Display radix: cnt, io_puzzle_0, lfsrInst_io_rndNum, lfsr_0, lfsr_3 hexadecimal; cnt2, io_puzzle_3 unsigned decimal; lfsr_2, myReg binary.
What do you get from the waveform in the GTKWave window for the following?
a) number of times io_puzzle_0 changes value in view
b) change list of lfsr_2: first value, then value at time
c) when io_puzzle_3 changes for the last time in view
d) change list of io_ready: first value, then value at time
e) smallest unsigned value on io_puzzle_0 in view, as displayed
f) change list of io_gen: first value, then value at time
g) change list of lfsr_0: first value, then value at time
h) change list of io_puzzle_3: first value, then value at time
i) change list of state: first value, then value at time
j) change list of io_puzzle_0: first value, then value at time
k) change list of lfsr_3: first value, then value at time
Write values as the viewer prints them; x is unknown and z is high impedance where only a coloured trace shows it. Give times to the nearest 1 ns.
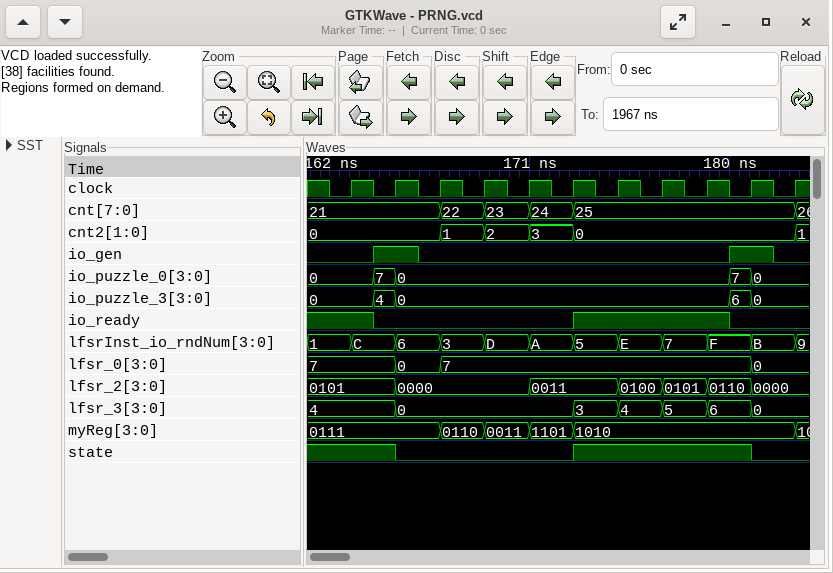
4
0101, 0000 at 165 ns, 0011 at 171 ns, 0100 at 175 ns, 0101 at 177 ns, 0110 at 179 ns, 0000 at 181 ns
181 ns
1, 0 at 164 ns, 1 at 173 ns, 0 at 180 ns
0
0, 1 at 164 ns, 0 at 166 ns, 1 at 180 ns, 0 at 182 ns
7, 0 at 165 ns, 7 at 167 ns, 0 at 181 ns
0, 4 at 164 ns, 0 at 165 ns, 6 at 180 ns, 0 at 181 ns
1, 0 at 165 ns, 1 at 173 ns, 0 at 181 ns
0, 7 at 164 ns, 0 at 165 ns, 7 at 180 ns, 0 at 181 ns
4, 0 at 165 ns, 3 at 173 ns, 4 at 175 ns, 5 at 177 ns, 6 at 179 ns, 0 at 181 ns
